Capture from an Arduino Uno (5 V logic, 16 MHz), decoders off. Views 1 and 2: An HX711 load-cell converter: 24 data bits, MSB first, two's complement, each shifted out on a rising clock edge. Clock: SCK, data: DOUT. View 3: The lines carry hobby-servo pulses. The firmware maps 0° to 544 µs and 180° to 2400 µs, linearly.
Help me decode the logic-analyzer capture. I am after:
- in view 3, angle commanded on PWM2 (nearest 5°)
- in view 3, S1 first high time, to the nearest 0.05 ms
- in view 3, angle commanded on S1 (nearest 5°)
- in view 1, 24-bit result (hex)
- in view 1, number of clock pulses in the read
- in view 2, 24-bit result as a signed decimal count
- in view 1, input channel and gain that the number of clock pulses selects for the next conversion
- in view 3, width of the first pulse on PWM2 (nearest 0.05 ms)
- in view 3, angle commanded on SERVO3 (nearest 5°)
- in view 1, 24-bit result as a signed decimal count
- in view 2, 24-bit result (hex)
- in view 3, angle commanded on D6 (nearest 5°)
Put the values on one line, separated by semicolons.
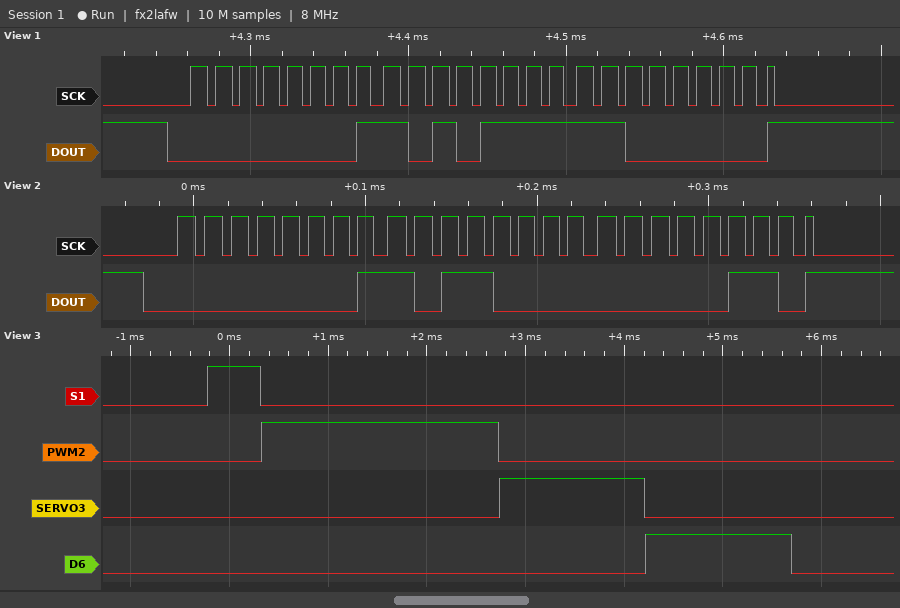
180°; 0.55 ms; 0°; 0x01AFC0; 25; 110598; channel A, gain 128; 2.40 ms; 90°; 110528; 0x01B006; 90°
